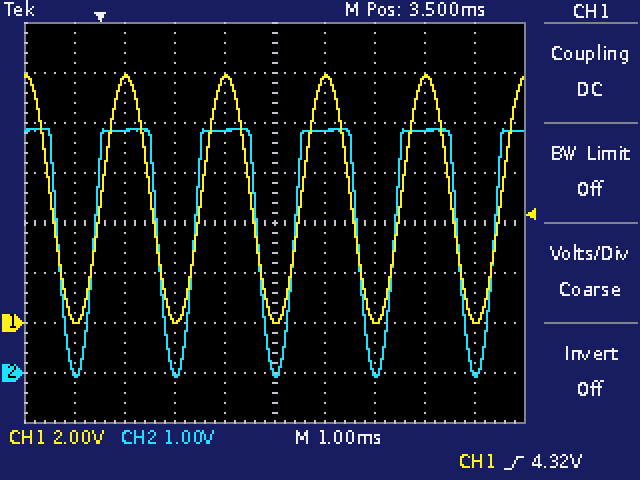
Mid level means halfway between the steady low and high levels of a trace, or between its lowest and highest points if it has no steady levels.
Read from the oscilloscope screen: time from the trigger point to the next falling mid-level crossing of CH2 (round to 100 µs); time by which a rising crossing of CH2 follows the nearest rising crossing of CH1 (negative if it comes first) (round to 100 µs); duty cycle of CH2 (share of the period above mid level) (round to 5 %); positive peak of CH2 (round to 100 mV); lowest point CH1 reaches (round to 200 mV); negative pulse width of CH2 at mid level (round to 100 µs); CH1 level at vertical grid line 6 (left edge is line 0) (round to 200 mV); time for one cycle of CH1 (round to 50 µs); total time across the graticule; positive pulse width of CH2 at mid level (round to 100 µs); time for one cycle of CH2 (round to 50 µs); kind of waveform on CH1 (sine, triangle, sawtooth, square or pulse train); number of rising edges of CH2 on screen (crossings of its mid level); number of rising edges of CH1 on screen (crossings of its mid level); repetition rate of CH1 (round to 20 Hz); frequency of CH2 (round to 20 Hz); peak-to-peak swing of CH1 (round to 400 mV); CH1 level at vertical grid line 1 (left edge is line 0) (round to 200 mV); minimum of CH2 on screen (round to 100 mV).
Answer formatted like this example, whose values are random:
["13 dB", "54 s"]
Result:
["1.2 ms", "-200 µs", "65 %", "4.9 V", "0.0 V", "700 µs", "9.8 V", "2.00 ms", "10 ms", "1.3 ms", "2.00 ms", "sine", "5", "5", "500 Hz", "500 Hz", "10.0 V", "200 mV", "-100 mV"]
